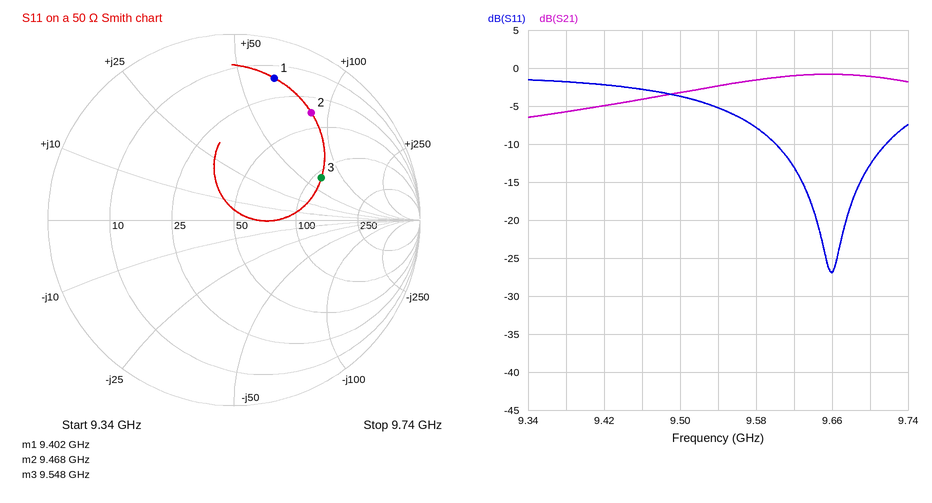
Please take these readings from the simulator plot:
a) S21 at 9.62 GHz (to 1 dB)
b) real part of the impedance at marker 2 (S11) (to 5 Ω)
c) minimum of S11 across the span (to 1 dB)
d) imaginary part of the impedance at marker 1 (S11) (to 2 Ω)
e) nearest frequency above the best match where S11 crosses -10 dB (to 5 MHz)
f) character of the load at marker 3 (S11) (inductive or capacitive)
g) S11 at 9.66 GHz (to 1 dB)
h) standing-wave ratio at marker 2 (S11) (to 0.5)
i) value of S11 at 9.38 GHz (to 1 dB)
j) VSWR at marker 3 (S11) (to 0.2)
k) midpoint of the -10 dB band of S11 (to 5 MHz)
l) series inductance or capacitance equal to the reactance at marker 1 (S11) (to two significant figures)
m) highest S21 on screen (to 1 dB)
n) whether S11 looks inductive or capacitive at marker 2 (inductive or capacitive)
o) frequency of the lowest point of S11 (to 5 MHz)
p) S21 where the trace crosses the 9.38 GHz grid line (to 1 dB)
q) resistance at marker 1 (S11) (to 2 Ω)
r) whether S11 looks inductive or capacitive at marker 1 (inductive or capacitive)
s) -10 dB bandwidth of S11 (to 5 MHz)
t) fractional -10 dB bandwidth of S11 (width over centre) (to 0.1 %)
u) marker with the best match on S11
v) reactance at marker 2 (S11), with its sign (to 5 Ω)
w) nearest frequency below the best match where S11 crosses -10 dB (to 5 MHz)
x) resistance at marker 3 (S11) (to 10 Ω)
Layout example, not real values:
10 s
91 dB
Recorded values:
-1 dB
35 Ω
-27 dB
+64 Ω
9.715 GHz
inductive
-27 dB
6.0
-2 dB
3.2
9.660 GHz
1.1 nH
-1 dB
inductive
9.660 GHz
-6 dB
16 Ω
inductive
115 MHz
1.2 %
marker 3
+85 Ω
9.600 GHz
110 Ω
